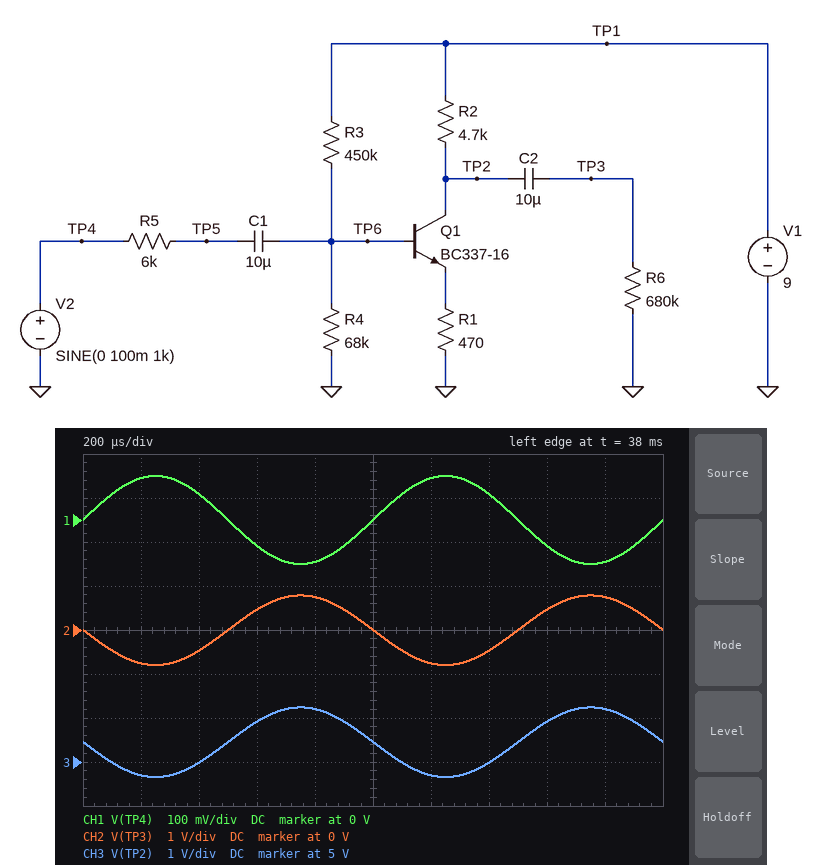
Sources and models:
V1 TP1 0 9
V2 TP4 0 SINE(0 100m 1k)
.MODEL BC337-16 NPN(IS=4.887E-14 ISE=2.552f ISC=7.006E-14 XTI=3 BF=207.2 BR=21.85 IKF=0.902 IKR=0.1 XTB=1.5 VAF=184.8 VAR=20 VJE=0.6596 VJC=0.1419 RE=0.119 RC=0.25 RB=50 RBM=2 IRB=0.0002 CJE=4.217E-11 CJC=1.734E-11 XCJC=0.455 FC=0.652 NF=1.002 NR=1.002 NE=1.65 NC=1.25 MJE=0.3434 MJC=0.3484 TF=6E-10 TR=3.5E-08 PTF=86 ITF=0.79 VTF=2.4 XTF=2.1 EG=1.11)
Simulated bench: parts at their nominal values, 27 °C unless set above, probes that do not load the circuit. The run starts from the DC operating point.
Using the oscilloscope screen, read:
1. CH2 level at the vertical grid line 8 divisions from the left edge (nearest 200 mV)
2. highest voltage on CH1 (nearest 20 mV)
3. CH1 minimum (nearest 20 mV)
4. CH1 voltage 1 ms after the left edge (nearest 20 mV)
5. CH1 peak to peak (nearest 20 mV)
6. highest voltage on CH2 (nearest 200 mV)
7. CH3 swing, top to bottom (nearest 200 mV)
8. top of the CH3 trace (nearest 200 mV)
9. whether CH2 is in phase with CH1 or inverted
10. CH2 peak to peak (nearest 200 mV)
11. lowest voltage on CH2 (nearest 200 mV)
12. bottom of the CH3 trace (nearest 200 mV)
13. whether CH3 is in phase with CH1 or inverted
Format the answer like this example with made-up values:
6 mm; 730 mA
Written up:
400 mV; 100 mV; -100 mV; 0 V; 200 mV; 800 mV; 1.6 V; 6.2 V; inverted; 1.6 V; -800 mV; 4.6 V; inverted
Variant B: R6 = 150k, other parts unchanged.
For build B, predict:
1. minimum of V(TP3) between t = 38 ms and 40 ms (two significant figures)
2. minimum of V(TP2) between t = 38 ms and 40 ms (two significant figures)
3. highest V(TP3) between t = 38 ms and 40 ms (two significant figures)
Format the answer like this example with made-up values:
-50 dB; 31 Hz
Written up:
-780 mV; 4.7 V; 770 mV
